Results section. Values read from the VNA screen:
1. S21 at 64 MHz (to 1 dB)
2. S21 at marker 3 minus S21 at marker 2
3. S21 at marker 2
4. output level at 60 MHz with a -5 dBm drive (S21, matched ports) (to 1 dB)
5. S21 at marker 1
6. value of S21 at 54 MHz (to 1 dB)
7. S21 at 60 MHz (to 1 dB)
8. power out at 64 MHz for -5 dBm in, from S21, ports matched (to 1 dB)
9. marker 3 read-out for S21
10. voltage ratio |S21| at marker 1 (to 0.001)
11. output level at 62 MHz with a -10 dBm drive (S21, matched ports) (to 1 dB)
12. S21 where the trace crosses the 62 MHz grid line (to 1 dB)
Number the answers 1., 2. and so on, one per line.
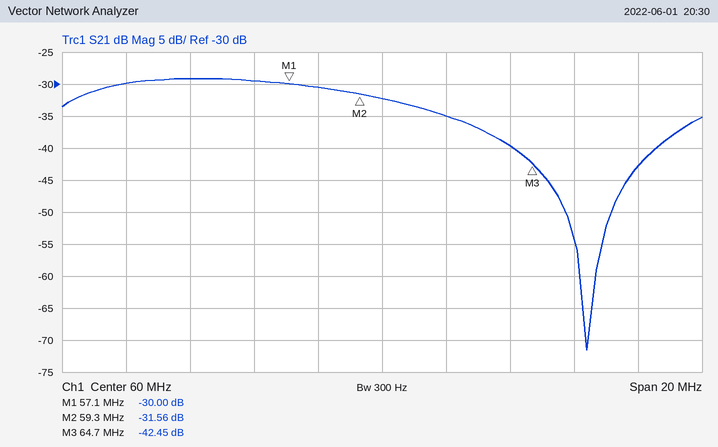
1. -40 dB
2. -10.89 dB
3. -31.56 dB
4. -37 dBm
5. -30.00 dB
6. -29 dB
7. -32 dB
8. -45 dBm
9. -42.45 dB
10. 0.032
11. -45 dBm
12. -35 dB
